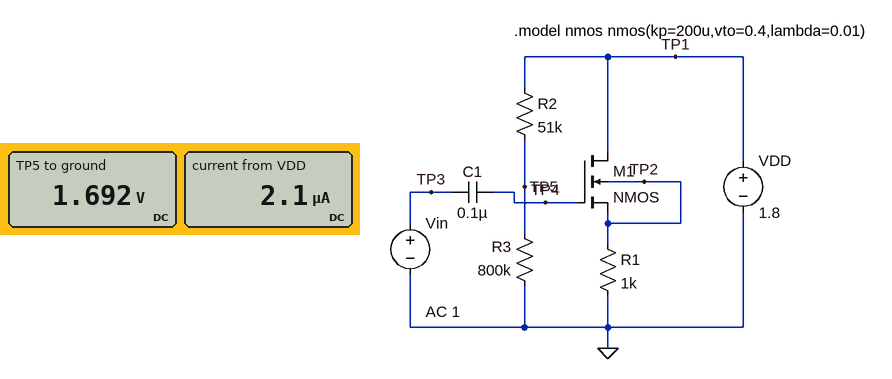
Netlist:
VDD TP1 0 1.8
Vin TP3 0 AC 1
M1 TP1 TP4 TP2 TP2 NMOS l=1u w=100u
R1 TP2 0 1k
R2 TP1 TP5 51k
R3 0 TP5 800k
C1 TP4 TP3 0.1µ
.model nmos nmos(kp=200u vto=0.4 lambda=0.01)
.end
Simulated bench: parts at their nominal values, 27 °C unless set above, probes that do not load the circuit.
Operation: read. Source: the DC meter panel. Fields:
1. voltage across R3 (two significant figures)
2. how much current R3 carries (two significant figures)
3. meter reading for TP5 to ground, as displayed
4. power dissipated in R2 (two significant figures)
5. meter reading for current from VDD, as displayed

1.7 V
2.1 µA
1.692 V
230 nW
2.1 µA
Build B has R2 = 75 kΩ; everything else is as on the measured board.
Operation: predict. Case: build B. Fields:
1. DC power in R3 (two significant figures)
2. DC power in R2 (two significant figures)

3.4 µW
320 nW
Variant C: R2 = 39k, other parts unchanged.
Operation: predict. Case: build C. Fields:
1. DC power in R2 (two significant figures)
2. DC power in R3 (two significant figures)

180 nW
3.7 µW
